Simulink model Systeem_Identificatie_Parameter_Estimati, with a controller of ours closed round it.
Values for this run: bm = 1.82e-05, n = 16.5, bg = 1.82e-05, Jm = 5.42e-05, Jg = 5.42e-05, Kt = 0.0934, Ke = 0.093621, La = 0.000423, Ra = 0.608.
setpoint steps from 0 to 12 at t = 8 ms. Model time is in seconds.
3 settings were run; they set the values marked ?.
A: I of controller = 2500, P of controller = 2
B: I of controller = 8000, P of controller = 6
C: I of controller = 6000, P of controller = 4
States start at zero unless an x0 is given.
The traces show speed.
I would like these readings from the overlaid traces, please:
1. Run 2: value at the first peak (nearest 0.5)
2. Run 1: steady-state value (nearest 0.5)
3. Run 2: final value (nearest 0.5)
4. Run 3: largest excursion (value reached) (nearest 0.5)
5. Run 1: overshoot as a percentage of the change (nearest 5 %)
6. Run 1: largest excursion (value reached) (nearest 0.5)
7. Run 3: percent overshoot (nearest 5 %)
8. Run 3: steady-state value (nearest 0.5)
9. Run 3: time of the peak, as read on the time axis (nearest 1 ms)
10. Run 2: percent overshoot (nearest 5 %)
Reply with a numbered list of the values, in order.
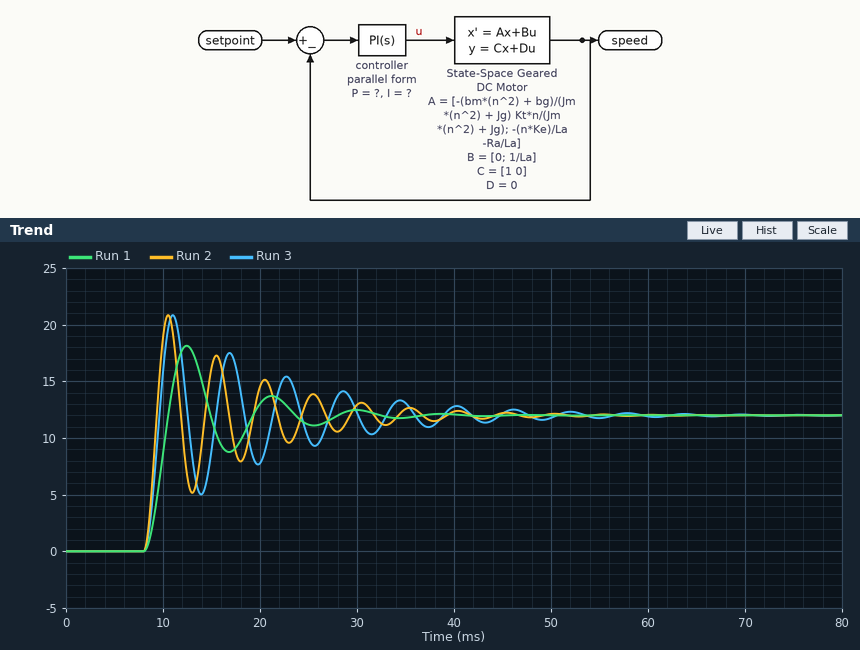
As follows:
1. 21.0
2. 12.0
3. 12.0
4. 21.0
5. 50 %
6. 18.0
7. 75 %
8. 12.0
9. 11 ms
10. 75 %
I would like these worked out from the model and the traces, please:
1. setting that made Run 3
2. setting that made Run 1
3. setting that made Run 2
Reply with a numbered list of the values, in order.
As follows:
1. C
2. A
3. B
